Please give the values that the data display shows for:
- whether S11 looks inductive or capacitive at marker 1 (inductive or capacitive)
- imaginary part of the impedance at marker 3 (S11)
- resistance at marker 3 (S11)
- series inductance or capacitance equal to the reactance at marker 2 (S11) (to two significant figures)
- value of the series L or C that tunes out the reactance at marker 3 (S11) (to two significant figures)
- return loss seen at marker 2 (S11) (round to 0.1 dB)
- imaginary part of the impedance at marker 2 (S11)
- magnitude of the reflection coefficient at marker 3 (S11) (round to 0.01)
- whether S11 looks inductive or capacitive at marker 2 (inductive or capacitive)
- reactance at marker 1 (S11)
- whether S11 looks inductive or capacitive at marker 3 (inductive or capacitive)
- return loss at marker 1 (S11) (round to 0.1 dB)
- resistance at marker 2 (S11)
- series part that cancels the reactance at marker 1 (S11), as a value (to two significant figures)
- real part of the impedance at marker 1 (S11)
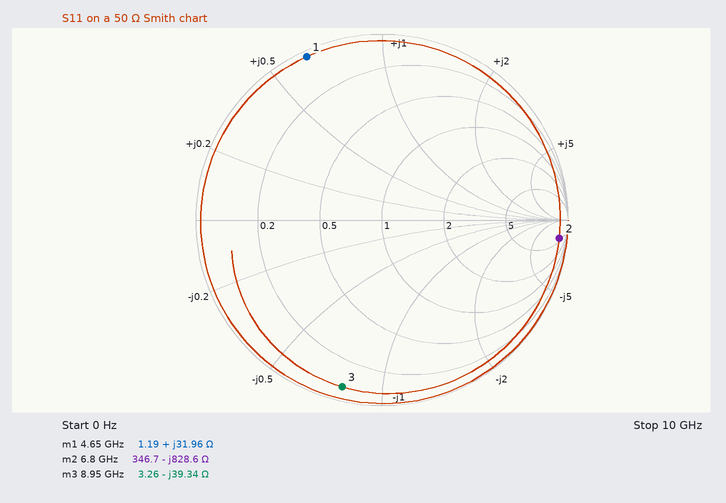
inductive
-39.34 Ω
3.26 Ω
28 fF
700 pH
0.4 dB
-828.6 Ω
0.92
capacitive
+31.96 Ω
capacitive
0.3 dB
346.7 Ω
1.1 pF
1.19 Ω
